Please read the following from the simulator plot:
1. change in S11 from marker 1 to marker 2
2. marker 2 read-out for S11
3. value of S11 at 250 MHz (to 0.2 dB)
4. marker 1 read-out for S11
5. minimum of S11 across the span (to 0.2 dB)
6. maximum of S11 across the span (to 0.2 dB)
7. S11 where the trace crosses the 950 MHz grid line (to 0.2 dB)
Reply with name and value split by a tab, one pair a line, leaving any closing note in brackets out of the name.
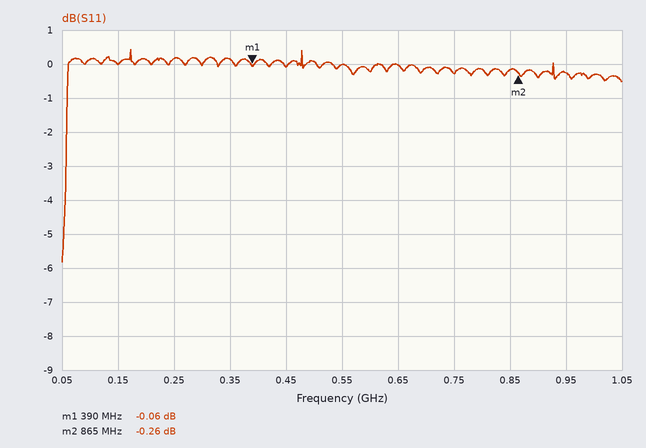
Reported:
change in S11 from marker 1 to marker 2	-0.20 dB
marker 2 read-out for S11	-0.26 dB
value of S11 at 250 MHz	0.2 dB
marker 1 read-out for S11	-0.06 dB
minimum of S11 across the span	-5.8 dB
maximum of S11 across the span	0.4 dB
S11 where the trace crosses the 950 MHz grid line	-0.2 dB
